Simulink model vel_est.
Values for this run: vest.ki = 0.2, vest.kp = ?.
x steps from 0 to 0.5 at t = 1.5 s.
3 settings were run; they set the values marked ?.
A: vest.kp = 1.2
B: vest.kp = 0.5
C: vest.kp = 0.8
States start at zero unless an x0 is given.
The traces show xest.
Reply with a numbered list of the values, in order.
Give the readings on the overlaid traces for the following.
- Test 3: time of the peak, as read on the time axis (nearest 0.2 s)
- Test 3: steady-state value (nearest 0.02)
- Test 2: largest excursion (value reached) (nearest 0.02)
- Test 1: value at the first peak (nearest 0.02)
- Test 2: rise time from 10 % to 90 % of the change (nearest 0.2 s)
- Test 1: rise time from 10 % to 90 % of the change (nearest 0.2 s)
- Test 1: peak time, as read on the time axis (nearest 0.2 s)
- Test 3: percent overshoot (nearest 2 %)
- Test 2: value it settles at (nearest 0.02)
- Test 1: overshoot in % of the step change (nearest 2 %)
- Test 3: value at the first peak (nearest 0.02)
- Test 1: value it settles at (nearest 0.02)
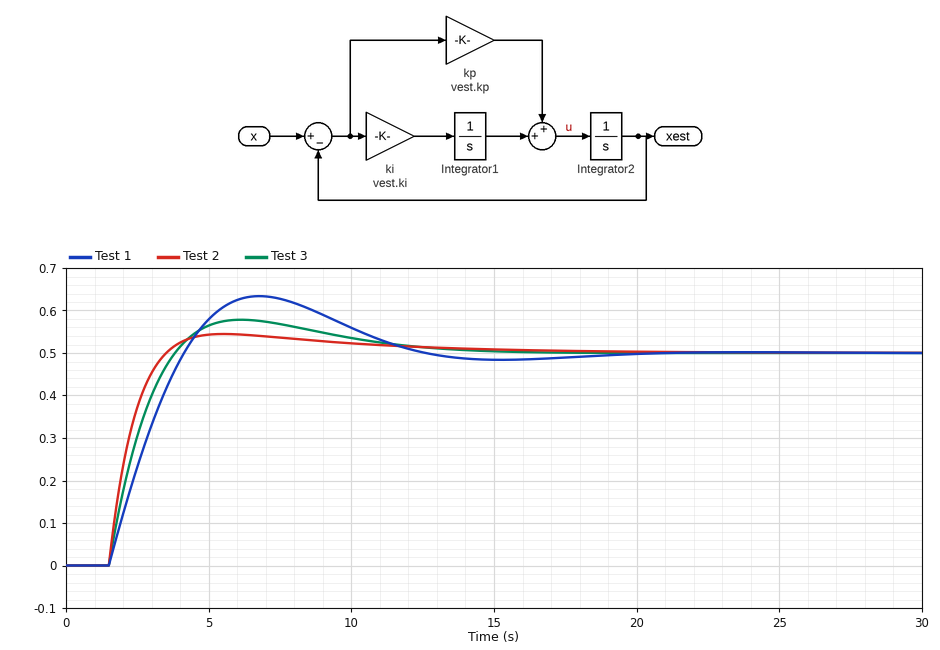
1. 6.2 s
2. 0.50
3. 0.54
4. 0.64
5. 1.4 s
6. 2.0 s
7. 6.8 s
8. 16 %
9. 0.50
10. 26 %
11. 0.58
12. 0.50
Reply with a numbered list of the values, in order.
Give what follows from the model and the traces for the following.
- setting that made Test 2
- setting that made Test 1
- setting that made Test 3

1. A
2. B
3. C
